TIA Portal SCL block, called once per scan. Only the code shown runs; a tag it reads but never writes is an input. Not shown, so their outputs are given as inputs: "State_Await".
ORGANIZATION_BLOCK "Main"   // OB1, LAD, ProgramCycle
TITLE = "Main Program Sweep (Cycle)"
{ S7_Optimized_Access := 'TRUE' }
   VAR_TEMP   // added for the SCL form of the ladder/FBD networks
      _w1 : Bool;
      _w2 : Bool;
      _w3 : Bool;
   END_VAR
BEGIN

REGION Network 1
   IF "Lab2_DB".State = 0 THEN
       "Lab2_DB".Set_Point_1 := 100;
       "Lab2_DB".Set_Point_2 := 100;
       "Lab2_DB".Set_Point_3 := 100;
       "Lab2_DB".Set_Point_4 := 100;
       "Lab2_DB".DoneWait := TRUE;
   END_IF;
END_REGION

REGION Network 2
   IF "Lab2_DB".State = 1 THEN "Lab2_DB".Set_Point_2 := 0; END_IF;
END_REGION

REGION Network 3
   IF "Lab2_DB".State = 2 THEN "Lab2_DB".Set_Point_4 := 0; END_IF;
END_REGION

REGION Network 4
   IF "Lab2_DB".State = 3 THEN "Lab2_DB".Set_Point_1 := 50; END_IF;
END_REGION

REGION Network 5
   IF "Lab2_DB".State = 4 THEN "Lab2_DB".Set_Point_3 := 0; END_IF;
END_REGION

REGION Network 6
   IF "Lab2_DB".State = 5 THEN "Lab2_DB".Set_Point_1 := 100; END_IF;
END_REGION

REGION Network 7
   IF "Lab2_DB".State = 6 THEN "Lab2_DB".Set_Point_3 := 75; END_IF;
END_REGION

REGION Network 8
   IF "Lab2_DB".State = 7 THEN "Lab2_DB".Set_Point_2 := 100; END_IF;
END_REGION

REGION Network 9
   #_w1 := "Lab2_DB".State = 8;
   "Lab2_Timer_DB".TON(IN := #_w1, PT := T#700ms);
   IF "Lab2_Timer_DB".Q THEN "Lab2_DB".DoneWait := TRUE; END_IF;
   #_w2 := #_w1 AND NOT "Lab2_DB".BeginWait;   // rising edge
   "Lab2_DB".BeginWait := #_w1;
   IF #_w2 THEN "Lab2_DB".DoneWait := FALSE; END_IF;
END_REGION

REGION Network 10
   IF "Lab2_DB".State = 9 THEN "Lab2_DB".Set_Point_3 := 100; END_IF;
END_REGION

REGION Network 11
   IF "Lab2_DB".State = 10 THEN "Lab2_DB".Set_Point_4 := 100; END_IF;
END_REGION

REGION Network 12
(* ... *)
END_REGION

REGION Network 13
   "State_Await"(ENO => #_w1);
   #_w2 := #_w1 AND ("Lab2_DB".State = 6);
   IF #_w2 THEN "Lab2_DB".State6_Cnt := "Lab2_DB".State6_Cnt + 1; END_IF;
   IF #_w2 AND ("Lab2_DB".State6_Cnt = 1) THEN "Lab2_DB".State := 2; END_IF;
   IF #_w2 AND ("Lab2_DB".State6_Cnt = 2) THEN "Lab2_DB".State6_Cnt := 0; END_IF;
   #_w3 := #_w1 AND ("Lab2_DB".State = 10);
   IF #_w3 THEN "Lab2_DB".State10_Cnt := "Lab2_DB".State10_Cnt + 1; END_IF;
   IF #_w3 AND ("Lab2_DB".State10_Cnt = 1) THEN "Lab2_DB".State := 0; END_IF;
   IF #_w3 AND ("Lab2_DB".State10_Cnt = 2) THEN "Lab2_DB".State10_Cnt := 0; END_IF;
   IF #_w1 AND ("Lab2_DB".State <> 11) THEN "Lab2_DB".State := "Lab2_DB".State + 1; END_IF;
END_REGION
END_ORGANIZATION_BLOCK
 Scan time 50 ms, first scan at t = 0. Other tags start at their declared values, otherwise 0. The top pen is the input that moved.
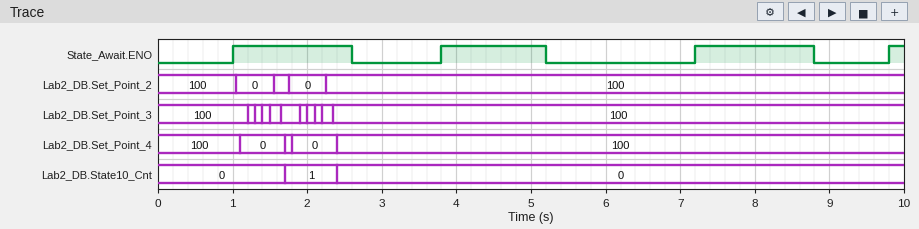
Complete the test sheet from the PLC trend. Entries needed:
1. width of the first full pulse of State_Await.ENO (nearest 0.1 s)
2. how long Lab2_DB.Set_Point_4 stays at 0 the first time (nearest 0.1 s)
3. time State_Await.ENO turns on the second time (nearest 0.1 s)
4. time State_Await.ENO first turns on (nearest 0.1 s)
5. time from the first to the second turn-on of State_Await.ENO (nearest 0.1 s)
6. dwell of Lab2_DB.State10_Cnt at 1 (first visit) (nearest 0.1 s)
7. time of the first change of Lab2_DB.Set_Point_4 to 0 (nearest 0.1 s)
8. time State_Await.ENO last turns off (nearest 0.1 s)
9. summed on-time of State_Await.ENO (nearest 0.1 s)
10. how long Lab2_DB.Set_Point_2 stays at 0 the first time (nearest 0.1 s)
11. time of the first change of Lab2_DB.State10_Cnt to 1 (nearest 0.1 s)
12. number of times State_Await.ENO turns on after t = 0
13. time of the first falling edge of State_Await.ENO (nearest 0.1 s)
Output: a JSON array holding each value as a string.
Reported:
["1.6 s", "0.6 s", "3.8 s", "1.0 s", "2.8 s", "0.7 s", "1.1 s", "8.8 s", "4.8 s", "0.5 s", "1.7 s", "4", "2.6 s"]
